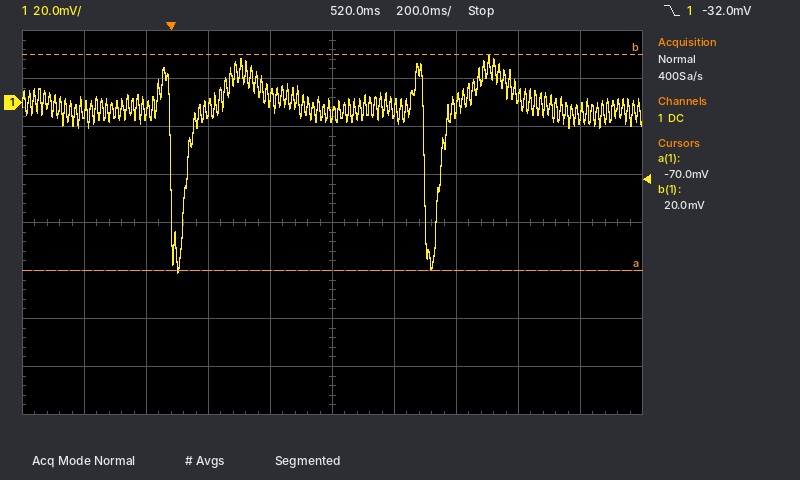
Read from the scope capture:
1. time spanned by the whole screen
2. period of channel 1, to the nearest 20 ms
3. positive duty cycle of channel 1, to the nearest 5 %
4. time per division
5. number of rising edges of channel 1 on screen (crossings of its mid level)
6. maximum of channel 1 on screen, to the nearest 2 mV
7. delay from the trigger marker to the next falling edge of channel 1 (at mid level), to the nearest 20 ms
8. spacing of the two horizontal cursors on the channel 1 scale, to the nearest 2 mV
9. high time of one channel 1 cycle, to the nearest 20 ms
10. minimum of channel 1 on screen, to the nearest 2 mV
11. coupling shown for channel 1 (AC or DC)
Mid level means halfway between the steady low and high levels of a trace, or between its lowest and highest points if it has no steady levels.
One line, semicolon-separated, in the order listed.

2 s; 820 ms; 95 %; 200 ms; 2; 20 mV; 820 ms; 90 mV; 760 ms; -70 mV; DC
